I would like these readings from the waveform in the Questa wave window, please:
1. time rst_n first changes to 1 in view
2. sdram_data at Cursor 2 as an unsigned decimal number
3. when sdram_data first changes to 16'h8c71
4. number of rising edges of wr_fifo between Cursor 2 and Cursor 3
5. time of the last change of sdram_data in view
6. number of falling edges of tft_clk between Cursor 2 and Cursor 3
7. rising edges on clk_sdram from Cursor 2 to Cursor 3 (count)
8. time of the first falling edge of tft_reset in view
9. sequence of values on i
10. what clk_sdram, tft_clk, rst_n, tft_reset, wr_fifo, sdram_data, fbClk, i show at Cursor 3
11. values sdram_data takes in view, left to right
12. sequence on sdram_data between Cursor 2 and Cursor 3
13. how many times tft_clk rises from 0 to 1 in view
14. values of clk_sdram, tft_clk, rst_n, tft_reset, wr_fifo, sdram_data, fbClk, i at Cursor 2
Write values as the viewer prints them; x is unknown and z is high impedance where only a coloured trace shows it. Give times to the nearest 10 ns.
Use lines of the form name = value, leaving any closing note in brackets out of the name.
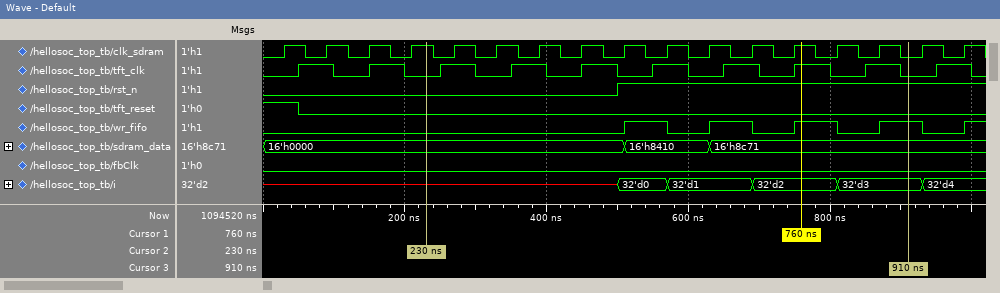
time rst_n first changes to 1 in view = 500 ns
sdram_data at Cursor 2 as an unsigned decimal number = 0
when sdram_data first changes to 16'h8c71 = 630 ns
number of rising edges of wr_fifo between Cursor 2 and Cursor 3 = 4
time of the last change of sdram_data in view = 630 ns
number of falling edges of tft_clk between Cursor 2 and Cursor 3 = 7
rising edges on clk_sdram from Cursor 2 to Cursor 3 = 11
time of the first falling edge of tft_reset in view = 50 ns
sequence of values on i = x, 32'd0, 32'd1, 32'd2, 32'd3, 32'd4
what clk_sdram, tft_clk, rst_n, tft_reset, wr_fifo, sdram_data, fbClk, i show at Cursor 3 = clk_sdram=0, tft_clk=0, rst_n=1, tft_reset=0, wr_fifo=1, sdram_data=16'h8c71, fbClk=0, i=32'd3
values sdram_data takes in view, left to right = 16'h0000, 16'h8410, 16'h8c71
sequence on sdram_data between Cursor 2 and Cursor 3 = 16'h0000, 16'h8410, 16'h8c71
how many times tft_clk rises from 0 to 1 in view = 10
values of clk_sdram, tft_clk, rst_n, tft_reset, wr_fifo, sdram_data, fbClk, i at Cursor 2 = clk_sdram=1, tft_clk=0, rst_n=0, tft_reset=0, wr_fifo=0, sdram_data=16'h0000, fbClk=0, i=x
